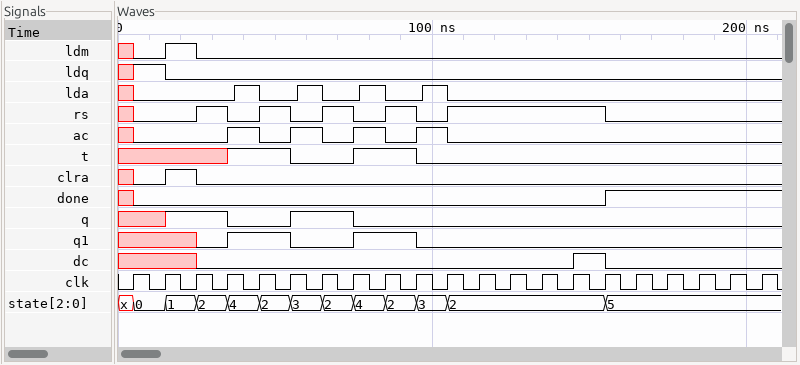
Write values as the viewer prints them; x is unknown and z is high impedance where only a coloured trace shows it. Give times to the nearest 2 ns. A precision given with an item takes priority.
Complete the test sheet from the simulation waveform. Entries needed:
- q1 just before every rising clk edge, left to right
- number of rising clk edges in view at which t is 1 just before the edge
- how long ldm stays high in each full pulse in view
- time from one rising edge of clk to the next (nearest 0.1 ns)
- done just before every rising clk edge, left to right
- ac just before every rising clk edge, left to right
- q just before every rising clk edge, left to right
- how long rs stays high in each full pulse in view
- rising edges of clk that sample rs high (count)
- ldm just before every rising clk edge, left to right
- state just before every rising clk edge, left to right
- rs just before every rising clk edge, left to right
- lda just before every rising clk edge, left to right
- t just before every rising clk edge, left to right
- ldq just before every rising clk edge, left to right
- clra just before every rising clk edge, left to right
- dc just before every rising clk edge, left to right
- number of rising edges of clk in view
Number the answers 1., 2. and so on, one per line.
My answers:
1. x x x 0 1 1 0 0 1 1 0 0 0 0 0 0 0 0 0 0 0
2. 4
3. 10 ns
4. 10 ns
5. x 0 0 0 0 0 0 0 0 0 0 0 0 0 0 0 1 1 1 1 1
6. x 0 0 0 1 0 1 0 1 0 1 0 0 0 0 0 0 0 0 0 0
7. x x 1 1 0 0 1 1 0 0 0 0 0 0 0 0 0 0 0 0 0
8. 10 ns, 10 ns, 10 ns, 10 ns, 50 ns
9. 9
10. x 0 1 0 0 0 0 0 0 0 0 0 0 0 0 0 0 0 0 0 0
11. x, 0, 1, 2, 4, 2, 3, 2, 4, 2, 3, 2, 2, 2, 2, 2, 5, 5, 5, 5, 5
12. x 0 0 1 0 1 0 1 0 1 0 1 1 1 1 1 0 0 0 0 0
13. x 0 0 0 1 0 1 0 1 0 1 0 0 0 0 0 0 0 0 0 0
14. x x x x 1 1 0 0 1 1 0 0 0 0 0 0 0 0 0 0 0
15. x 1 0 0 0 0 0 0 0 0 0 0 0 0 0 0 0 0 0 0 0
16. x 0 1 0 0 0 0 0 0 0 0 0 0 0 0 0 0 0 0 0 0
17. x x x 0 0 0 0 0 0 0 0 0 0 0 0 1 0 0 0 0 0
18. 21
